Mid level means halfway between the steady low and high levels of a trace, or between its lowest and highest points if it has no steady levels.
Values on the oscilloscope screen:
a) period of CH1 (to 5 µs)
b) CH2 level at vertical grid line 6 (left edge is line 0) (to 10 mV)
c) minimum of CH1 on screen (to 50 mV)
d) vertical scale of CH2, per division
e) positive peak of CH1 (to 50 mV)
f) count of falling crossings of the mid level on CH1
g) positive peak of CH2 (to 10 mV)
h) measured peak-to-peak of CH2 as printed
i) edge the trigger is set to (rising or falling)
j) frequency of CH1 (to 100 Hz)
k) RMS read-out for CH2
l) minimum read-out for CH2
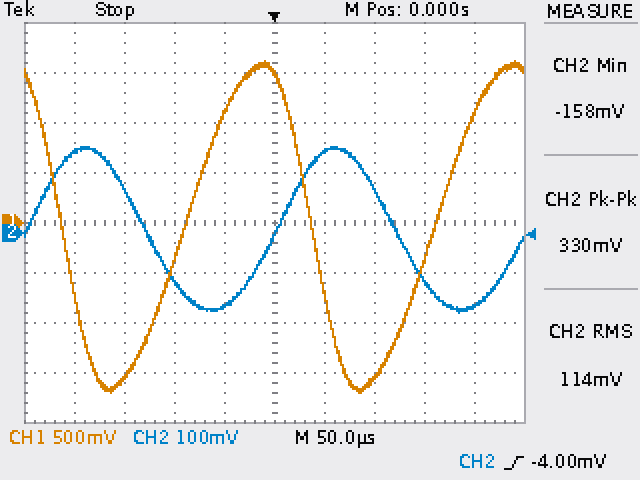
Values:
250 µs
160 mV
-1.70 V
100 mV
1.60 V
2
170 mV
330 mV
rising
4.0 kHz
114 mV
-158 mV
